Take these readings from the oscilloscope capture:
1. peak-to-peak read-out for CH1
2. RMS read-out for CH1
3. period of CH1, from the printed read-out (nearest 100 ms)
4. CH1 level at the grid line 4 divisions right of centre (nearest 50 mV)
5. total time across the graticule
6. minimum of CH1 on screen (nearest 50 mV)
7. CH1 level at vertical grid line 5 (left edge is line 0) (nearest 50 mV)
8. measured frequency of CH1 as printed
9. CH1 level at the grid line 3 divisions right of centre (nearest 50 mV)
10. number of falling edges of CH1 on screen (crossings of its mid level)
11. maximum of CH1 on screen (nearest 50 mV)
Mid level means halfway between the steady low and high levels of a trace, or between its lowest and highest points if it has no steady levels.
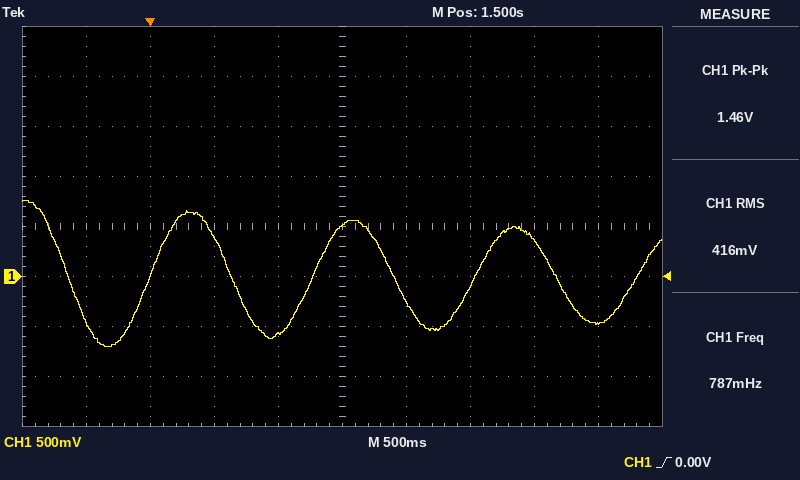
1.46 V
416 mV
1.3 s
-450 mV
5 s
-700 mV
500 mV
787 mHz
350 mV
4
750 mV
